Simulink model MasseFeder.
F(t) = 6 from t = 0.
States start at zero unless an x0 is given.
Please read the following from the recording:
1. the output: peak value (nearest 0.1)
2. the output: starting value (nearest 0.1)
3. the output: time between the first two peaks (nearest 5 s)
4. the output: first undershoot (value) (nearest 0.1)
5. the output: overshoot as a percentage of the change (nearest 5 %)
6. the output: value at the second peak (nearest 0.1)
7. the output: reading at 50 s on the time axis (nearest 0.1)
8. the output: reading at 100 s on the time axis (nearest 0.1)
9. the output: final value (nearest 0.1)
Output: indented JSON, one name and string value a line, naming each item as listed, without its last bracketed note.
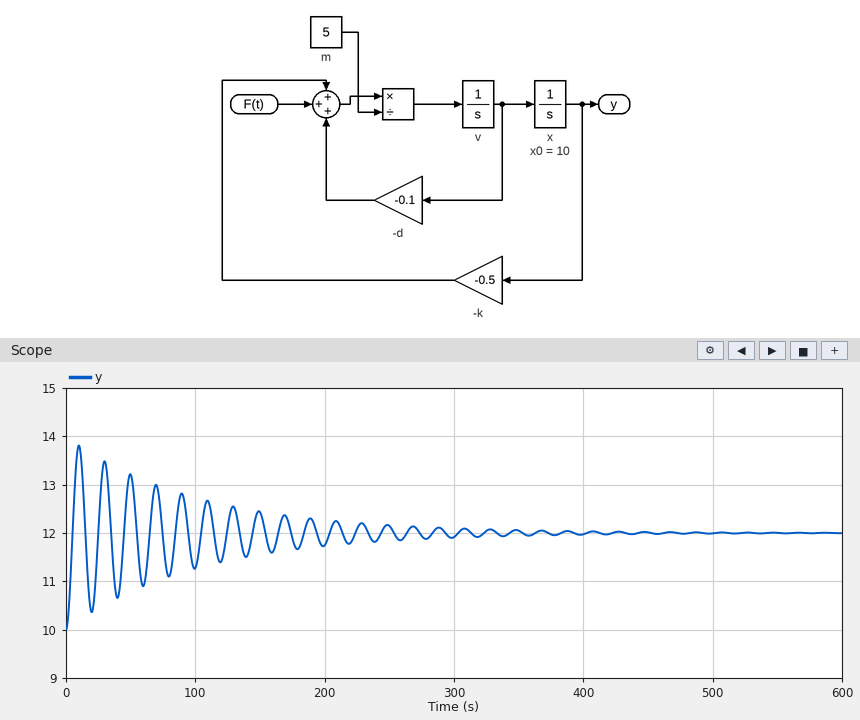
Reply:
{
  "the output: peak value": "13.8",
  "the output: starting value": "10.0",
  "the output: time between the first two peaks": "20 s",
  "the output: first undershoot (value)": "10.4",
  "the output: overshoot as a percentage of the change": "90 %",
  "the output: value at the second peak": "13.5",
  "the output: reading at 50 s on the time axis": "13.2",
  "the output: reading at 100 s on the time axis": "11.3",
  "the output: final value": "12.0"
}
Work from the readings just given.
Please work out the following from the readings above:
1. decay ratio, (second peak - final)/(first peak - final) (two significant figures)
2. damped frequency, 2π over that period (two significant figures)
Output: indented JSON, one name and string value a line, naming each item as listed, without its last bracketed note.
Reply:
{
  "decay ratio, (second peak - final)/(first peak - final)": "0.83",
  "damped frequency, 2π over that period": "0.31 rad/s"
}
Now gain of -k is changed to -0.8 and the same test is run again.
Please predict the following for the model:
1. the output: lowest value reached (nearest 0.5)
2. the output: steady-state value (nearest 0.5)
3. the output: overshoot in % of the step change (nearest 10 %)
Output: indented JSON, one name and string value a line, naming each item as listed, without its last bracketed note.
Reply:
{
  "the output: lowest value reached": "5.0",
  "the output: steady-state value": "7.5",
  "the output: overshoot in % of the step change": "90 %"
}
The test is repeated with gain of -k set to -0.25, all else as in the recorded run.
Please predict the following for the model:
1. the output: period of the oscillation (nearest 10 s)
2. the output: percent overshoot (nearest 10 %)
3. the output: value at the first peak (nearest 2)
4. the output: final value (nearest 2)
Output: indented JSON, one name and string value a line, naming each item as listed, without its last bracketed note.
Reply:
{
  "the output: period of the oscillation": "30 s",
  "the output: percent overshoot": "90 %",
  "the output: value at the first peak": "36",
  "the output: final value": "24"
}
